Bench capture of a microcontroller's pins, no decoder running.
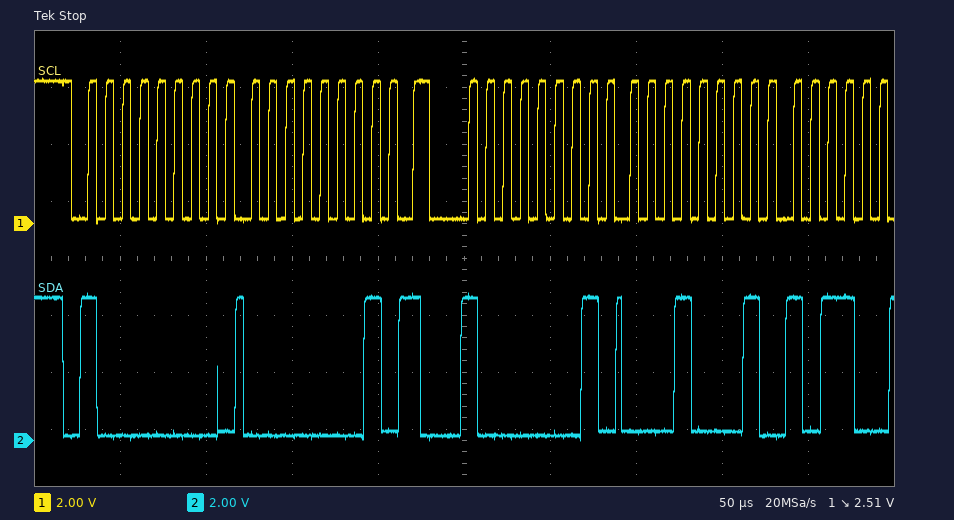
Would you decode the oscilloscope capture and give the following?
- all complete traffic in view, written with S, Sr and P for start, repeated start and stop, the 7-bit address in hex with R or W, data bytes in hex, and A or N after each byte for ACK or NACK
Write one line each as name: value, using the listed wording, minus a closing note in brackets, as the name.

all complete traffic in view, written with S, Sr and P for start, repeated start and stop, the 7-bit address in hex with R or W, data bytes in hex, and A or N after each byte for ACK or NACK: S 40W A 01 A Sr 40R A 11 A
